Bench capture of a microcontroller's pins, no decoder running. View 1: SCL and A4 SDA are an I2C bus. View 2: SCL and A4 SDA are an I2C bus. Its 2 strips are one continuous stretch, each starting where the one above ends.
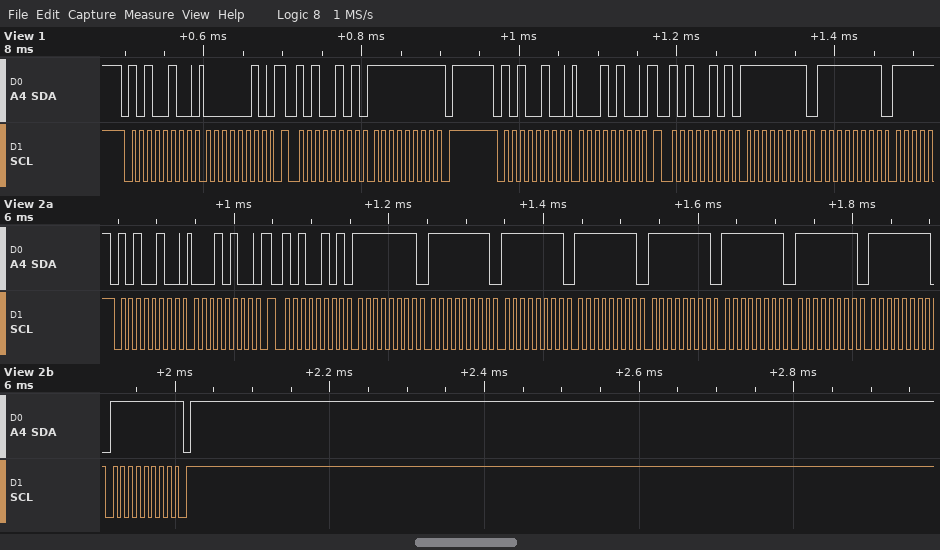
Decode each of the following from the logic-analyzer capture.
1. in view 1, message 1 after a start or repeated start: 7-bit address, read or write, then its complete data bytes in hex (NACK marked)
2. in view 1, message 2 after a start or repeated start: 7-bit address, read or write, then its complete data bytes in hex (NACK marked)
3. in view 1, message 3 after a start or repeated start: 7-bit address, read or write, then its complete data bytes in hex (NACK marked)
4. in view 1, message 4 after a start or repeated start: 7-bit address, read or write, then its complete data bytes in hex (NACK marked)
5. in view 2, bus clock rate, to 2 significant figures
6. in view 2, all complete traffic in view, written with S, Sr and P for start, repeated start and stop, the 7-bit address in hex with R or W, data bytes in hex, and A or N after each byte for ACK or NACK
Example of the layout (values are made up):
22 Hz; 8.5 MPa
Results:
0x52 write: 02; 0x52 read: FF NACK; 0x52 write: 14; 0x52 read: FF FF; 100 kHz; S 52W A 14 A Sr 52R A FF A FF A FF A FF A FF A FF A FF A FF A FF N P
